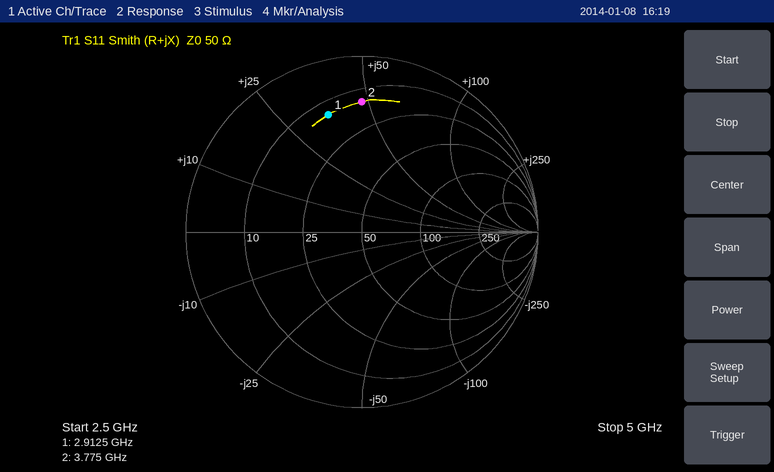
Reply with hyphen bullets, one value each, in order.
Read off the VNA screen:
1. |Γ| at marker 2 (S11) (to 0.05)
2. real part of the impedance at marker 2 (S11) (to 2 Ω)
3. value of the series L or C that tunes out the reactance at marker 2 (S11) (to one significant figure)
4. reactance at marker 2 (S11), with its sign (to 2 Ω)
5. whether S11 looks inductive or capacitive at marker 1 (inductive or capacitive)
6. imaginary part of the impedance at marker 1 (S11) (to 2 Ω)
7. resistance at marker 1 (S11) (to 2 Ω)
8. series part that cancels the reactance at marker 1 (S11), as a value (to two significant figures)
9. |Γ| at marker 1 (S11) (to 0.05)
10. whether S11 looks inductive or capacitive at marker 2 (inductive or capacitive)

- 0.75
- 14 Ω
- 900 fF
- +48 Ω
- inductive
- +36 Ω
- 14 Ω
- 1.5 pF
- 0.70
- inductive
